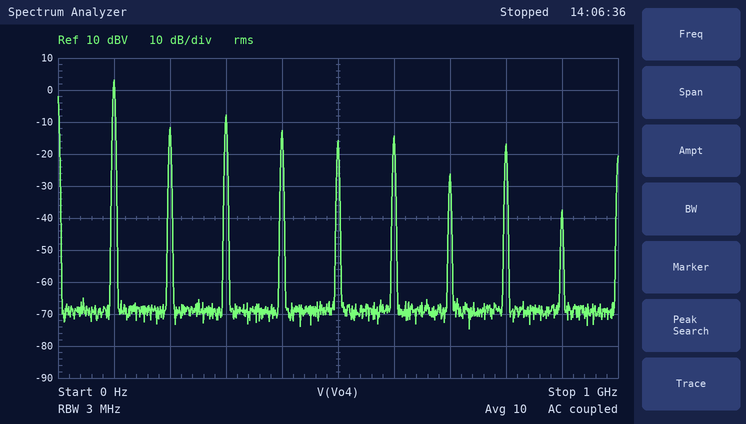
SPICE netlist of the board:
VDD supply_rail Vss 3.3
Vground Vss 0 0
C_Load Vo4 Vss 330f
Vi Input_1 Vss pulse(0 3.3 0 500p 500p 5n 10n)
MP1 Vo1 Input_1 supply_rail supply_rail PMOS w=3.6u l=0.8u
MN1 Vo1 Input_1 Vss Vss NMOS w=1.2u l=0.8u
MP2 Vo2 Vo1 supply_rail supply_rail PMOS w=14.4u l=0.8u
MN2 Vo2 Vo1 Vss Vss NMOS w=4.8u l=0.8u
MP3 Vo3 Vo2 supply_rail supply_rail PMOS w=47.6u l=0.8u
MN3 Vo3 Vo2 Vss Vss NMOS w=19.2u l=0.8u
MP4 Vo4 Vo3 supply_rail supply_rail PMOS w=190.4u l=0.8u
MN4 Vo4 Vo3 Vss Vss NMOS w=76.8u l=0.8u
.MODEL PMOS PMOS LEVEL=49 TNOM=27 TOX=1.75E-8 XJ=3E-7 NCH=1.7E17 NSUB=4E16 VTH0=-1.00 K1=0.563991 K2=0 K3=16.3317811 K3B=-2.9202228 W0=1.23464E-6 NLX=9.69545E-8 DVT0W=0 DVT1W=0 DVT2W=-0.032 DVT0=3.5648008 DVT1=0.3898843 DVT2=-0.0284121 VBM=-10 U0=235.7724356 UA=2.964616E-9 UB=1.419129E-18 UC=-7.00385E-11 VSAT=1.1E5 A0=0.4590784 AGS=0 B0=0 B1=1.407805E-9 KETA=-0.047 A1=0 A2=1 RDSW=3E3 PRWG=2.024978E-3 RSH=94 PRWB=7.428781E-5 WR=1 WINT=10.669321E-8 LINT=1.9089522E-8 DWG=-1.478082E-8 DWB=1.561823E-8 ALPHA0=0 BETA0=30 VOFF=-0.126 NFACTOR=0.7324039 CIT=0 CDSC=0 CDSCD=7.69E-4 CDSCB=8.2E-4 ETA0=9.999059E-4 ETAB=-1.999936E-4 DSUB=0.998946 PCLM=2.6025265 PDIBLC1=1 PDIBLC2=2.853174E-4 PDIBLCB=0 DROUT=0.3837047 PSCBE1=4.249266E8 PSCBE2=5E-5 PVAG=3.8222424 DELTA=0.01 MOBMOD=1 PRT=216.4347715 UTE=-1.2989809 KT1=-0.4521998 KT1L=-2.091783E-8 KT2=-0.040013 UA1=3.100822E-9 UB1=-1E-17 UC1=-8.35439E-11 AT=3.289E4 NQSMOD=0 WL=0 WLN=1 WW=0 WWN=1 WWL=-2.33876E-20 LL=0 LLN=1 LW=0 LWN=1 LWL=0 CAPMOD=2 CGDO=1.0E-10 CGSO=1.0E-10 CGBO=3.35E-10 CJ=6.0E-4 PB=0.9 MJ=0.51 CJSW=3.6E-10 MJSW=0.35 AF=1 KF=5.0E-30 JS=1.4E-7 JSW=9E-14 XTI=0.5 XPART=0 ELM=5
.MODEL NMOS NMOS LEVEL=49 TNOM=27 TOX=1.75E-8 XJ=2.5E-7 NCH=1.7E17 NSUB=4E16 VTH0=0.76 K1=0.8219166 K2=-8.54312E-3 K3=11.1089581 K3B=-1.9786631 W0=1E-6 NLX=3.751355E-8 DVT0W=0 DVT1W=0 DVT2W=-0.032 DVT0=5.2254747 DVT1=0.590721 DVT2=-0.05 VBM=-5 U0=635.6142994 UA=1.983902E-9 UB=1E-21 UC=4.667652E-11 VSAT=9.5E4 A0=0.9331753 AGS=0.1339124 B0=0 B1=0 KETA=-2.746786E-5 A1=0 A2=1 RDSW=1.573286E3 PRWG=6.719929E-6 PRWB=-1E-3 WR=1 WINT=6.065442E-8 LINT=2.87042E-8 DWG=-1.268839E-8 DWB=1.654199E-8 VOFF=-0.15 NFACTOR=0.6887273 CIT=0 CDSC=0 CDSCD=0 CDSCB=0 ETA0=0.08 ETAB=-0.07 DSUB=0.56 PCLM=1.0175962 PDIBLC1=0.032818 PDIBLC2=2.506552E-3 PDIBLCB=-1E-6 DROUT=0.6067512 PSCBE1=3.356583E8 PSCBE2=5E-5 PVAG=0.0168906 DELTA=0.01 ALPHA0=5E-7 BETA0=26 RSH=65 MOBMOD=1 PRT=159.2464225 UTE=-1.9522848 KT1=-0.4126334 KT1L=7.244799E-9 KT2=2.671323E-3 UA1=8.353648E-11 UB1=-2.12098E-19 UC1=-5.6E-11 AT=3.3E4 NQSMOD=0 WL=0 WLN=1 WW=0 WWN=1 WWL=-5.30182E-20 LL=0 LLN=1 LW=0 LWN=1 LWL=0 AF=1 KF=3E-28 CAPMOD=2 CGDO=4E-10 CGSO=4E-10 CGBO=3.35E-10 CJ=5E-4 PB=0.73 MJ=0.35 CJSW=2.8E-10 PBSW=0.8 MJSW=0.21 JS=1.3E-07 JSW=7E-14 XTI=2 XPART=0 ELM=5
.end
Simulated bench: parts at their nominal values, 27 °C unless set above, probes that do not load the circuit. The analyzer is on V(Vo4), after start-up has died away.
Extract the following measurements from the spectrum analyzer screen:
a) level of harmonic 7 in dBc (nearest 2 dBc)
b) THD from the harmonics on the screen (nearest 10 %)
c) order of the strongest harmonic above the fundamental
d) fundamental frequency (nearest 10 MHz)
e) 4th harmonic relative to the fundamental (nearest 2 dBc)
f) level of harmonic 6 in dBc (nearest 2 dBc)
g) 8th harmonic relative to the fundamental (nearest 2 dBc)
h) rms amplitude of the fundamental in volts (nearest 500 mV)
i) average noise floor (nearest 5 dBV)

-30 dBc
40 %
3
100 MHz
-16 dBc
-18 dBc
-20 dBc
1.5 V
-70 dBV
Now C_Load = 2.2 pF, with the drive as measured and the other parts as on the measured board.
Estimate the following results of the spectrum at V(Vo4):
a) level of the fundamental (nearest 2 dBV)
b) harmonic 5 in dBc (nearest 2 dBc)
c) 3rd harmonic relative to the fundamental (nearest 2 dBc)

2 dBV
-26 dBc
-14 dBc
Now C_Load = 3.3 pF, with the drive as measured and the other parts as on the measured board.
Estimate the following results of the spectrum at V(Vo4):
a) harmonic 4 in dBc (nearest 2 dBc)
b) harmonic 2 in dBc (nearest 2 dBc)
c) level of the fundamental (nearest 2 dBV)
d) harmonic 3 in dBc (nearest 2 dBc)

-24 dBc
-18 dBc
2 dBV
-16 dBc
